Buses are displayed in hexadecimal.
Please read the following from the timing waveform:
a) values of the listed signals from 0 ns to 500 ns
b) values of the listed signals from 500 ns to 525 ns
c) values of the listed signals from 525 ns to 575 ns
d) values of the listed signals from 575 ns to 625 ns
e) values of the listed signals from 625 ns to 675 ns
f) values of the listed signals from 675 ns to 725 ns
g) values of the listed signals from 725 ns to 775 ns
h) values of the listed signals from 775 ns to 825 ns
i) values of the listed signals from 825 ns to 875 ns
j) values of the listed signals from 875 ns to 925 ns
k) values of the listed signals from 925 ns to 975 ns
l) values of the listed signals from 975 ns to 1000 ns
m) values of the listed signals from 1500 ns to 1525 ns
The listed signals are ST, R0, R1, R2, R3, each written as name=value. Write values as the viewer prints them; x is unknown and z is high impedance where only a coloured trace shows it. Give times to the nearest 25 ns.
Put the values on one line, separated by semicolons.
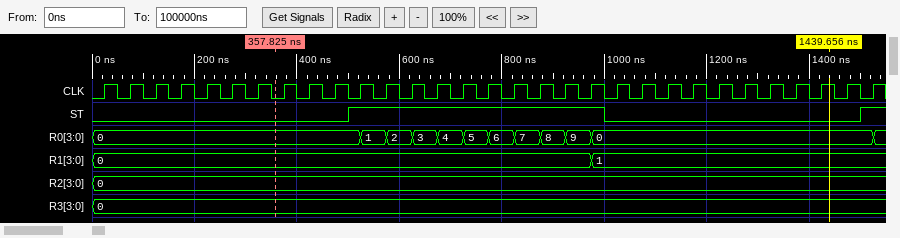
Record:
ST=0, R0=0, R1=0, R2=0, R3=0; ST=1, R0=0, R1=0, R2=0, R3=0; ST=1, R0=1, R1=0, R2=0, R3=0; ST=1, R0=2, R1=0, R2=0, R3=0; ST=1, R0=3, R1=0, R2=0, R3=0; ST=1, R0=4, R1=0, R2=0, R3=0; ST=1, R0=5, R1=0, R2=0, R3=0; ST=1, R0=6, R1=0, R2=0, R3=0; ST=1, R0=7, R1=0, R2=0, R3=0; ST=1, R0=8, R1=0, R2=0, R3=0; ST=1, R0=9, R1=0, R2=0, R3=0; ST=1, R0=0, R1=1, R2=0, R3=0; ST=1, R0=0, R1=1, R2=0, R3=0
